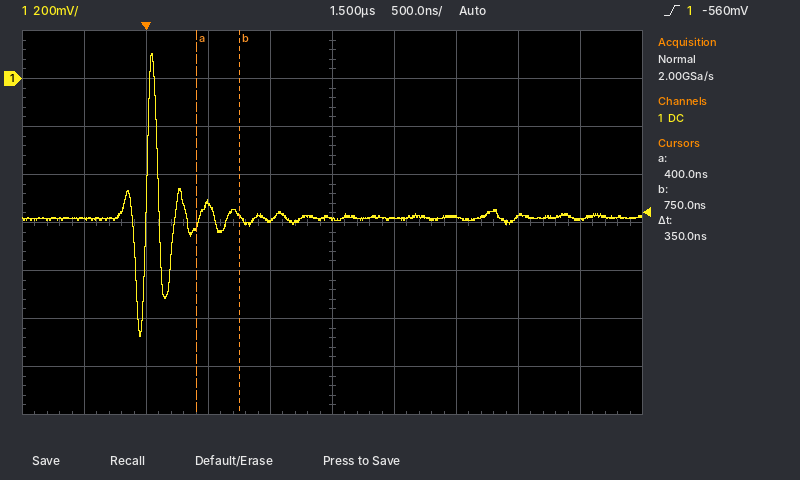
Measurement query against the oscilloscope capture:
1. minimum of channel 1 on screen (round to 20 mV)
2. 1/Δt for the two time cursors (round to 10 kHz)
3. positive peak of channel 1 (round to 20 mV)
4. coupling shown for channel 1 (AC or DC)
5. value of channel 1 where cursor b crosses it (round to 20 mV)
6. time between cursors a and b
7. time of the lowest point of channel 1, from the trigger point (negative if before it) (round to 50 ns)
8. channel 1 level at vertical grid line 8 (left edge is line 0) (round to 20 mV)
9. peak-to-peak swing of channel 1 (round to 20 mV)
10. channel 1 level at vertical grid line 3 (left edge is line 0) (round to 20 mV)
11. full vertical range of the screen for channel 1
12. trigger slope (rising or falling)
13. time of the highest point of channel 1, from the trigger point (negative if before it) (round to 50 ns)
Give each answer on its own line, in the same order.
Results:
-1.08 V
2.86 MHz
100 mV
DC
-580 mV
350 ns
-50 ns
-580 mV
1.18 V
-520 mV
1.6 V
rising
+50 ns
